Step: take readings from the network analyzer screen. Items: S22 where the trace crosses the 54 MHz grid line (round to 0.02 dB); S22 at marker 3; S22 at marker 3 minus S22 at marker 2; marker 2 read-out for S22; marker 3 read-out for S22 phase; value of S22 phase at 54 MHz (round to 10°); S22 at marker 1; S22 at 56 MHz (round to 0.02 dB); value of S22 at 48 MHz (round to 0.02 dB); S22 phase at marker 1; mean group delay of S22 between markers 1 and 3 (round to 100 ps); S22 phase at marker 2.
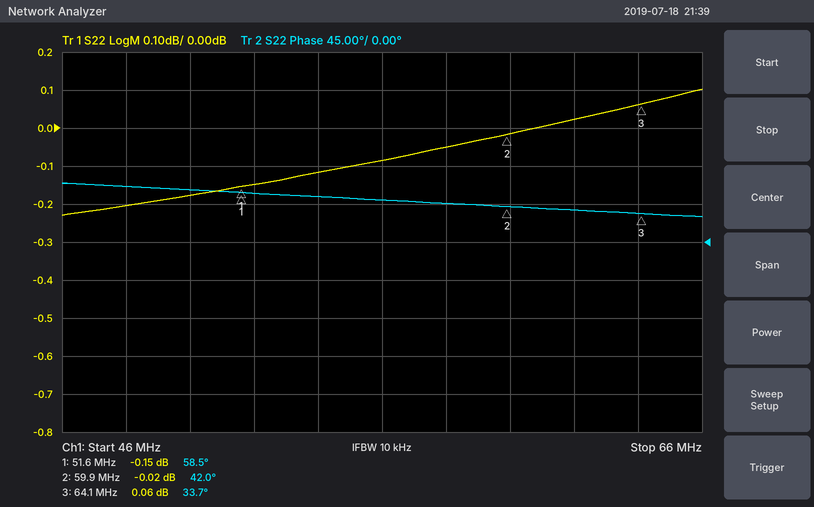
-0.12 dB
0.06 dB
0.08 dB
-0.02 dB
33.7°
50°
-0.15 dB
-0.08 dB
-0.20 dB
58.5°
5.5 ns
42.0°
